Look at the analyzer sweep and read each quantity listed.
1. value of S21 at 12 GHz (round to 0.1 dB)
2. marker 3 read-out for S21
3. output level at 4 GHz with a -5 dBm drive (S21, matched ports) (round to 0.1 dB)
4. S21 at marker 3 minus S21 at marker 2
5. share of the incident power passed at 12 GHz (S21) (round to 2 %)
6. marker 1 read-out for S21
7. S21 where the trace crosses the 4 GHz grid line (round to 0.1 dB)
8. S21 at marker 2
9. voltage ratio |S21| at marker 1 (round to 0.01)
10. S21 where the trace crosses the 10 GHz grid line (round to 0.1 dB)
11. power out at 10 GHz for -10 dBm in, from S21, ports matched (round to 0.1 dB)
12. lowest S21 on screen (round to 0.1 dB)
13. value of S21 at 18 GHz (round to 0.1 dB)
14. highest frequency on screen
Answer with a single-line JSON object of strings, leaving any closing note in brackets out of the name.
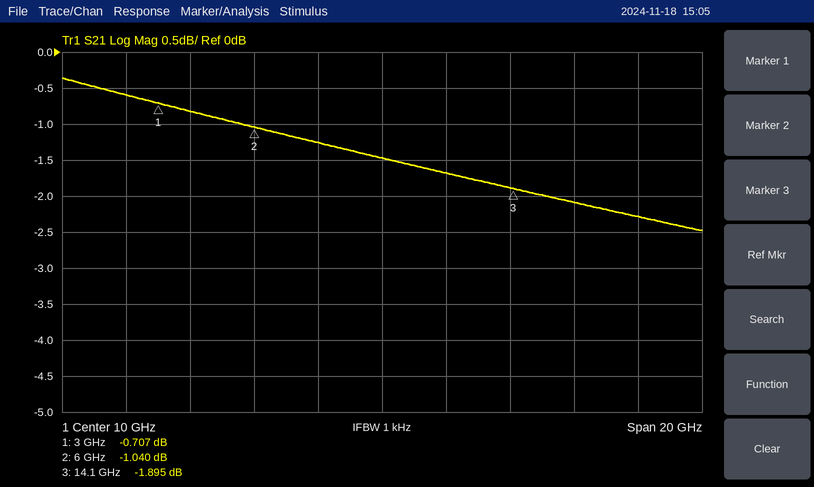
{"value of S21 at 12 GHz": "-1.7 dB", "marker 3 read-out for S21": "-1.895 dB", "output level at 4 GHz with a -5 dBm drive (S21, matched ports)": "-5.8 dBm", "S21 at marker 3 minus S21 at marker 2": "-0.855 dB", "share of the incident power passed at 12 GHz (S21)": "68 %", "marker 1 read-out for S21": "-0.707 dB", "S21 where the trace crosses the 4 GHz grid line": "-0.8 dB", "S21 at marker 2": "-1.040 dB", "voltage ratio |S21| at marker 1": "0.92", "S21 where the trace crosses the 10 GHz grid line": "-1.5 dB", "power out at 10 GHz for -10 dBm in, from S21, ports matched": "-11.5 dBm", "lowest S21 on screen": "-2.5 dB", "value of S21 at 18 GHz": "-2.3 dB", "highest frequency on screen": "20 GHz"}
